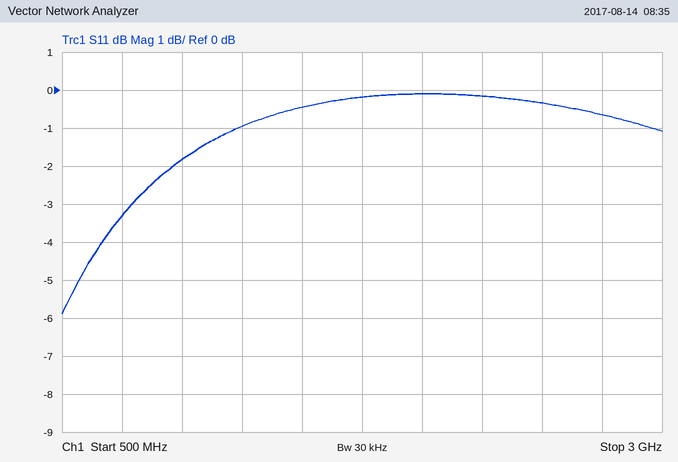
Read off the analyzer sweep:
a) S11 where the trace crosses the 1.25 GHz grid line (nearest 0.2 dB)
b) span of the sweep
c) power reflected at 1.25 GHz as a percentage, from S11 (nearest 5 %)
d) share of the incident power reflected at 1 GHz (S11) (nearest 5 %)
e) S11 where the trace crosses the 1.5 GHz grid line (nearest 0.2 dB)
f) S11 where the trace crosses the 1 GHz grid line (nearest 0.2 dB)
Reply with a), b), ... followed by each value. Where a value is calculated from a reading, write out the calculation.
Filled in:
a) -1.0 dB
b) 2.5 GHz
c) 10^(-1/10) ≈ 79.4 %, so 80 % to the nearest 5 %
d) 10^(-1.8/10) ≈ 66.1 %, so 65 % to the nearest 5 %
e) -0.4 dB
f) -1.8 dB
